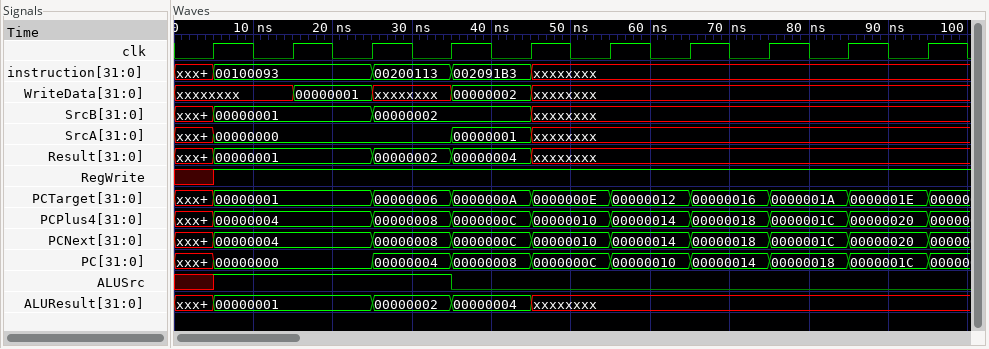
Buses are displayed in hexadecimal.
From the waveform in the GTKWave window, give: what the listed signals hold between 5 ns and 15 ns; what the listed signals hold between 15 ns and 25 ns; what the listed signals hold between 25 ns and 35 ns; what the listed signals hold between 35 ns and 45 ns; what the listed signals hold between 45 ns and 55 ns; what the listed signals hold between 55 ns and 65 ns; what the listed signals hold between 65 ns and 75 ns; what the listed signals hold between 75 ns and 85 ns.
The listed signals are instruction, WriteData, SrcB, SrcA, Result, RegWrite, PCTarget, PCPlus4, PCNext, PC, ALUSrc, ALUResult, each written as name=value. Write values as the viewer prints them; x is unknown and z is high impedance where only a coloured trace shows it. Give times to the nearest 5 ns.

instruction=00100093, WriteData=xxxxxxxx, SrcB=00000001, SrcA=00000000, Result=00000001, RegWrite=1, PCTarget=00000001, PCPlus4=00000004, PCNext=00000004, PC=00000000, ALUSrc=1, ALUResult=00000001
instruction=00100093, WriteData=00000001, SrcB=00000001, SrcA=00000000, Result=00000001, RegWrite=1, PCTarget=00000001, PCPlus4=00000004, PCNext=00000004, PC=00000000, ALUSrc=1, ALUResult=00000001
instruction=00200113, WriteData=xxxxxxxx, SrcB=00000002, SrcA=00000000, Result=00000002, RegWrite=1, PCTarget=00000006, PCPlus4=00000008, PCNext=00000008, PC=00000004, ALUSrc=1, ALUResult=00000002
instruction=002091B3, WriteData=00000002, SrcB=00000002, SrcA=00000001, Result=00000004, RegWrite=1, PCTarget=0000000A, PCPlus4=0000000C, PCNext=0000000C, PC=00000008, ALUSrc=0, ALUResult=00000004
instruction=xxxxxxxx, WriteData=xxxxxxxx, SrcB=xxxxxxxx, SrcA=xxxxxxxx, Result=xxxxxxxx, RegWrite=1, PCTarget=0000000E, PCPlus4=00000010, PCNext=00000010, PC=0000000C, ALUSrc=0, ALUResult=xxxxxxxx
instruction=xxxxxxxx, WriteData=xxxxxxxx, SrcB=xxxxxxxx, SrcA=xxxxxxxx, Result=xxxxxxxx, RegWrite=1, PCTarget=00000012, PCPlus4=00000014, PCNext=00000014, PC=00000010, ALUSrc=0, ALUResult=xxxxxxxx
instruction=xxxxxxxx, WriteData=xxxxxxxx, SrcB=xxxxxxxx, SrcA=xxxxxxxx, Result=xxxxxxxx, RegWrite=1, PCTarget=00000016, PCPlus4=00000018, PCNext=00000018, PC=00000014, ALUSrc=0, ALUResult=xxxxxxxx
instruction=xxxxxxxx, WriteData=xxxxxxxx, SrcB=xxxxxxxx, SrcA=xxxxxxxx, Result=xxxxxxxx, RegWrite=1, PCTarget=0000001A, PCPlus4=0000001C, PCNext=0000001C, PC=00000018, ALUSrc=0, ALUResult=xxxxxxxx
